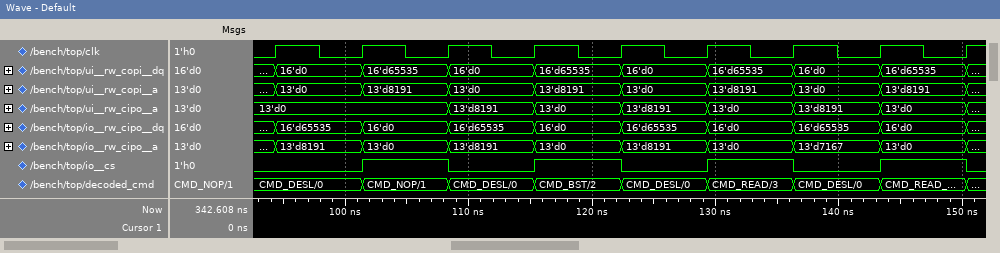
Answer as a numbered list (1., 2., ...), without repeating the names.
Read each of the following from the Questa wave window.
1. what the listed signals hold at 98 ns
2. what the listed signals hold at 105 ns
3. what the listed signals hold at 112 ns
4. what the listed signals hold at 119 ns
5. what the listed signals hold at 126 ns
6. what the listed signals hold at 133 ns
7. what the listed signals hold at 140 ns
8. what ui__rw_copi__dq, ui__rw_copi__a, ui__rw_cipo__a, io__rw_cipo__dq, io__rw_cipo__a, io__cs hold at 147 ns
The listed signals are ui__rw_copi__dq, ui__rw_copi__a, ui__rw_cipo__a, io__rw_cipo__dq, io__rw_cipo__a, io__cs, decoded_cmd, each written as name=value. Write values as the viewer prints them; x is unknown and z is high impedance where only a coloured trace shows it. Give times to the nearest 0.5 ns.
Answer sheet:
1. ui__rw_copi__dq=16'd0, ui__rw_copi__a=13'd0, ui__rw_cipo__a=13'd0, io__rw_cipo__dq=16'd65535, io__rw_cipo__a=13'd8191, io__cs=0, decoded_cmd=CMD_DESL/0
2. ui__rw_copi__dq=16'd65535, ui__rw_copi__a=13'd8191, ui__rw_cipo__a=13'd0, io__rw_cipo__dq=16'd0, io__rw_cipo__a=13'd0, io__cs=1, decoded_cmd=CMD_NOP/1
3. ui__rw_copi__dq=16'd0, ui__rw_copi__a=13'd0, ui__rw_cipo__a=13'd8191, io__rw_cipo__dq=16'd65535, io__rw_cipo__a=13'd8191, io__cs=0, decoded_cmd=CMD_DESL/0
4. ui__rw_copi__dq=16'd65535, ui__rw_copi__a=13'd8191, ui__rw_cipo__a=13'd0, io__rw_cipo__dq=16'd0, io__rw_cipo__a=13'd0, io__cs=1, decoded_cmd=CMD_BST/2
5. ui__rw_copi__dq=16'd0, ui__rw_copi__a=13'd0, ui__rw_cipo__a=13'd8191, io__rw_cipo__dq=16'd65535, io__rw_cipo__a=13'd8191, io__cs=0, decoded_cmd=CMD_DESL/0
6. ui__rw_copi__dq=16'd65535, ui__rw_copi__a=13'd8191, ui__rw_cipo__a=13'd0, io__rw_cipo__dq=16'd0, io__rw_cipo__a=13'd0, io__cs=1, decoded_cmd=CMD_READ/3
7. ui__rw_copi__dq=16'd0, ui__rw_copi__a=13'd0, ui__rw_cipo__a=13'd8191, io__rw_cipo__dq=16'd65535, io__rw_cipo__a=13'd7167, io__cs=0, decoded_cmd=CMD_DESL/0
8. ui__rw_copi__dq=16'd65535, ui__rw_copi__a=13'd8191, ui__rw_cipo__a=13'd0, io__rw_cipo__dq=16'd0, io__rw_cipo__a=13'd0, io__cs=1
